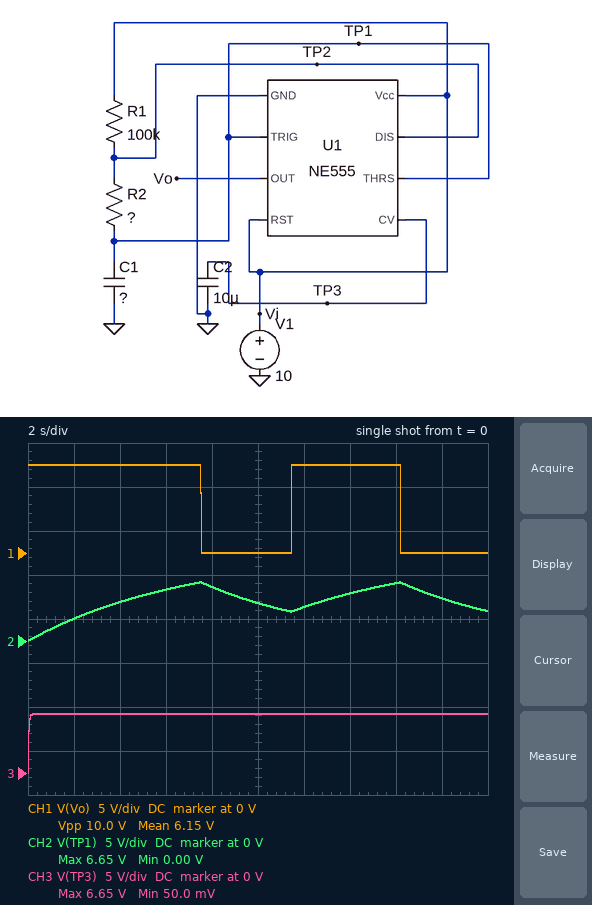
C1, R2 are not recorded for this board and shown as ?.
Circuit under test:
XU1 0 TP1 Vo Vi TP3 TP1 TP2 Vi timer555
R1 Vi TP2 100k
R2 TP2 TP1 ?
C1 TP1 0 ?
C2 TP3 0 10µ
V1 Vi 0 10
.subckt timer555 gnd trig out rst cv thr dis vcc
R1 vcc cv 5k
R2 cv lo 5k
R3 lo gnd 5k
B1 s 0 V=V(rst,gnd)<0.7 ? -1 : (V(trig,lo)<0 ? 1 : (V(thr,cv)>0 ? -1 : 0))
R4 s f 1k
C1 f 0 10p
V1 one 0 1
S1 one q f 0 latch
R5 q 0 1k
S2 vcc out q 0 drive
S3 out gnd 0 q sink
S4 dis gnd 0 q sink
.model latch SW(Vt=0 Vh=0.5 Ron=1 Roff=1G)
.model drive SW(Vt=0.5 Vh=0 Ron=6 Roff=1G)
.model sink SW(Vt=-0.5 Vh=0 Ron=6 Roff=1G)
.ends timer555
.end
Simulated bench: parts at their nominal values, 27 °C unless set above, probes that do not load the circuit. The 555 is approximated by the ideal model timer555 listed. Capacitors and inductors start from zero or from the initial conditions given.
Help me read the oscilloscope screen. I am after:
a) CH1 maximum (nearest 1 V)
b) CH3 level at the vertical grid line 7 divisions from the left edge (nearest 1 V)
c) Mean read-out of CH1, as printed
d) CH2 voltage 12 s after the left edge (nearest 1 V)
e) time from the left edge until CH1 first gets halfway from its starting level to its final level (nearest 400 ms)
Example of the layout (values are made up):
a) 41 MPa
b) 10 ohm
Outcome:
a) 10 V
b) 7 V
c) 6.15 V
d) 4 V
e) 7.6 s
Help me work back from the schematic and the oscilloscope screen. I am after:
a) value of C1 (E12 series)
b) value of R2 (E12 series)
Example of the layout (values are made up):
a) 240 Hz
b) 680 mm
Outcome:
a) 12 µF
b) 470 kΩ
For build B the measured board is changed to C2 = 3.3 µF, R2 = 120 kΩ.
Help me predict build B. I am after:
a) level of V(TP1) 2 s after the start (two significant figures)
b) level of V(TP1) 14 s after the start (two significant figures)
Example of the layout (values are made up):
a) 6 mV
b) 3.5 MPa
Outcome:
a) 5.3 V
b) 6.4 V
